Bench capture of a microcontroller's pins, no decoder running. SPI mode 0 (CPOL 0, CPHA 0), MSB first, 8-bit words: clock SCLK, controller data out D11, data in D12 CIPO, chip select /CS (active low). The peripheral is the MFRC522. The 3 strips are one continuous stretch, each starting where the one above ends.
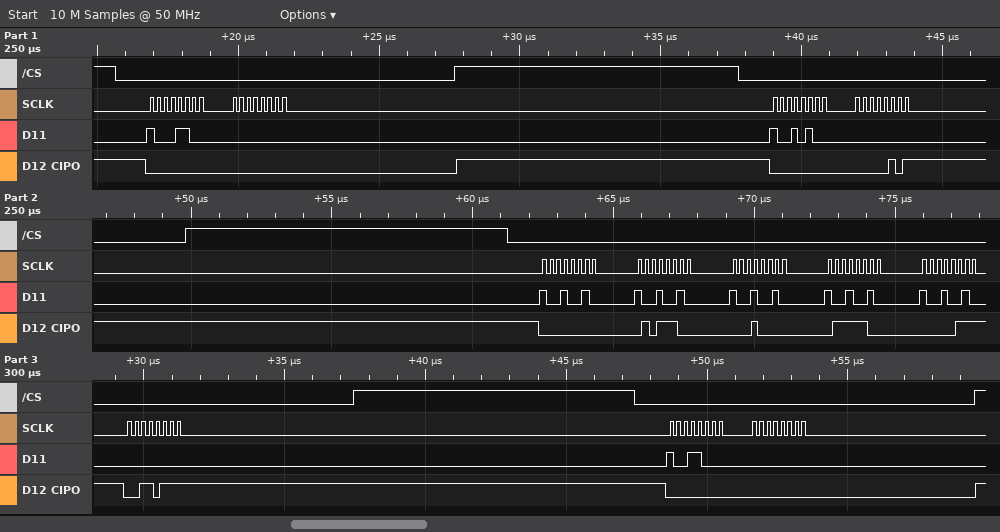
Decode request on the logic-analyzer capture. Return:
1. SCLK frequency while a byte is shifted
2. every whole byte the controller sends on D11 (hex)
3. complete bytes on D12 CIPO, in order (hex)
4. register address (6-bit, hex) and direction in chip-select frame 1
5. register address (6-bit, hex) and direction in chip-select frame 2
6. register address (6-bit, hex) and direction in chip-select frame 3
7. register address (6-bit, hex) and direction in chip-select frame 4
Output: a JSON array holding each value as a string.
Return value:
["4 MHz", "8C 00 94 00 92 92 92 92 92 00 98 00", "00 00 00 05 00 5C 10 7C 07 37 00 00", "0x06 read", "0x0A read", "0x09 read", "0x0C read"]
